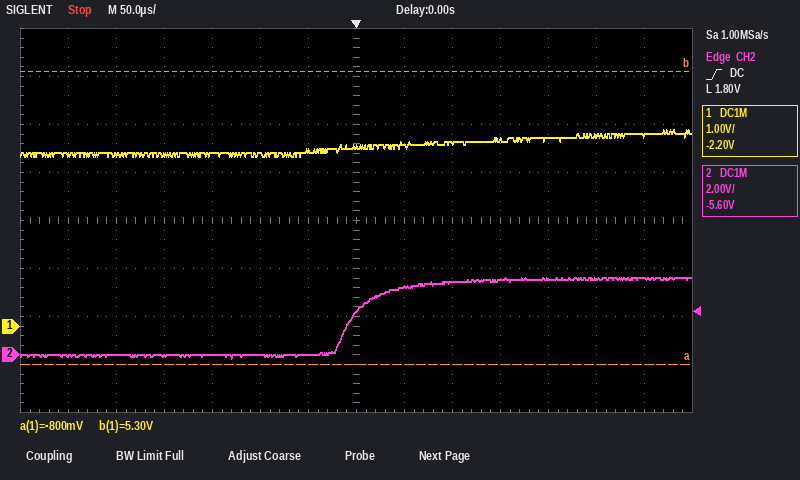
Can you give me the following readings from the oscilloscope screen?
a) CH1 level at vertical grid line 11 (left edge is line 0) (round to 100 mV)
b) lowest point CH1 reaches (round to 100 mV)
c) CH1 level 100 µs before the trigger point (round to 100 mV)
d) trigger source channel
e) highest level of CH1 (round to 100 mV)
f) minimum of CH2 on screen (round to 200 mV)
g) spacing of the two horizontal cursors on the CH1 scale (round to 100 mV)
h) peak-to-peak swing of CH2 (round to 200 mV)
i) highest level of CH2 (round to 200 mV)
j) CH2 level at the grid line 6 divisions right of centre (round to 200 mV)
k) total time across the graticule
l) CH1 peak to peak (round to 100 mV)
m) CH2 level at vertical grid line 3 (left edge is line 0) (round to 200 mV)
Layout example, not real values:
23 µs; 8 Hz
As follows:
3.9 V; 3.5 V; 3.6 V; CH2; 4.1 V; -200 mV; 6.1 V; 3.4 V; 3.2 V; 3.2 V; 700 µs; 600 mV; 0.0 V
